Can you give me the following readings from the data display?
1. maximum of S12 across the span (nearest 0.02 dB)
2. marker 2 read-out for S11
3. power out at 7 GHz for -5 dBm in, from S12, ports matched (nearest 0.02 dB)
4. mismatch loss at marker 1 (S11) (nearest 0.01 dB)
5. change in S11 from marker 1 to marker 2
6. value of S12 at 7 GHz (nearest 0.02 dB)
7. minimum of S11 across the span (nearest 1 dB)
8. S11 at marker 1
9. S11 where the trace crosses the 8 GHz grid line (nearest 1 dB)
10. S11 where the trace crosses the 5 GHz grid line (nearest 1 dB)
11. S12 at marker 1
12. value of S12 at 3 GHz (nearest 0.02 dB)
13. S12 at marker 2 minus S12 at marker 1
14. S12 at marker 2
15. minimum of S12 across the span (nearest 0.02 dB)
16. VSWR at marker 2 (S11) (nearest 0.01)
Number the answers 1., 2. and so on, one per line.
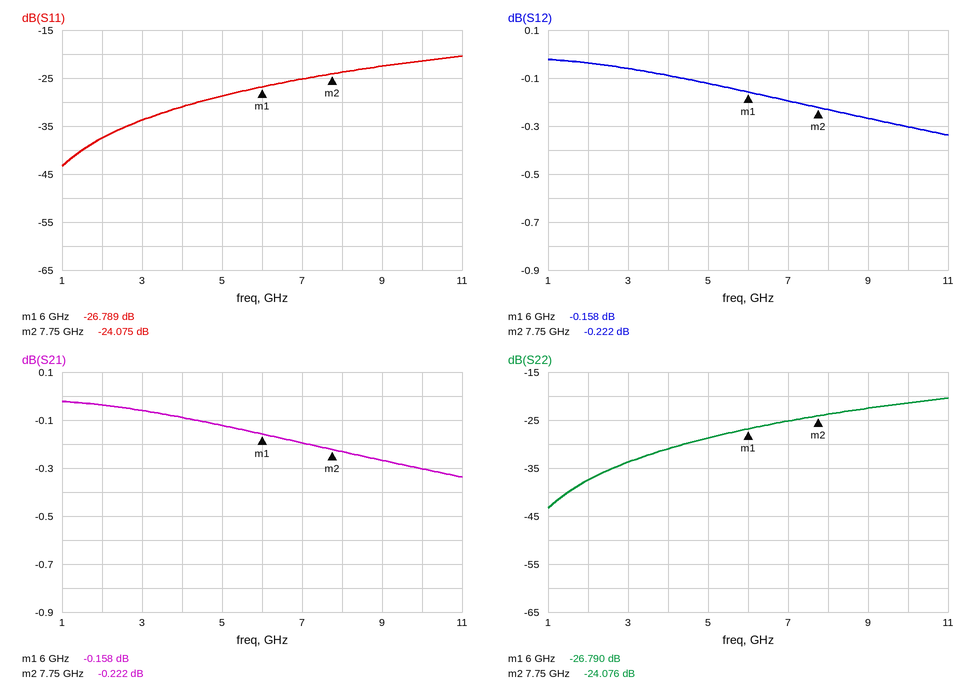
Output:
1. -0.02 dB
2. -24.075 dB
3. -5.20 dBm
4. 0.01 dB
5. 2.714 dB
6. -0.20 dB
7. -43 dB
8. -26.789 dB
9. -24 dB
10. -29 dB
11. -0.158 dB
12. -0.06 dB
13. -0.064 dB
14. -0.222 dB
15. -0.34 dB
16. 1.13
